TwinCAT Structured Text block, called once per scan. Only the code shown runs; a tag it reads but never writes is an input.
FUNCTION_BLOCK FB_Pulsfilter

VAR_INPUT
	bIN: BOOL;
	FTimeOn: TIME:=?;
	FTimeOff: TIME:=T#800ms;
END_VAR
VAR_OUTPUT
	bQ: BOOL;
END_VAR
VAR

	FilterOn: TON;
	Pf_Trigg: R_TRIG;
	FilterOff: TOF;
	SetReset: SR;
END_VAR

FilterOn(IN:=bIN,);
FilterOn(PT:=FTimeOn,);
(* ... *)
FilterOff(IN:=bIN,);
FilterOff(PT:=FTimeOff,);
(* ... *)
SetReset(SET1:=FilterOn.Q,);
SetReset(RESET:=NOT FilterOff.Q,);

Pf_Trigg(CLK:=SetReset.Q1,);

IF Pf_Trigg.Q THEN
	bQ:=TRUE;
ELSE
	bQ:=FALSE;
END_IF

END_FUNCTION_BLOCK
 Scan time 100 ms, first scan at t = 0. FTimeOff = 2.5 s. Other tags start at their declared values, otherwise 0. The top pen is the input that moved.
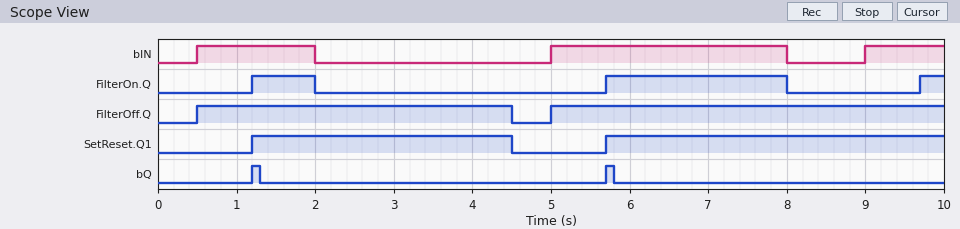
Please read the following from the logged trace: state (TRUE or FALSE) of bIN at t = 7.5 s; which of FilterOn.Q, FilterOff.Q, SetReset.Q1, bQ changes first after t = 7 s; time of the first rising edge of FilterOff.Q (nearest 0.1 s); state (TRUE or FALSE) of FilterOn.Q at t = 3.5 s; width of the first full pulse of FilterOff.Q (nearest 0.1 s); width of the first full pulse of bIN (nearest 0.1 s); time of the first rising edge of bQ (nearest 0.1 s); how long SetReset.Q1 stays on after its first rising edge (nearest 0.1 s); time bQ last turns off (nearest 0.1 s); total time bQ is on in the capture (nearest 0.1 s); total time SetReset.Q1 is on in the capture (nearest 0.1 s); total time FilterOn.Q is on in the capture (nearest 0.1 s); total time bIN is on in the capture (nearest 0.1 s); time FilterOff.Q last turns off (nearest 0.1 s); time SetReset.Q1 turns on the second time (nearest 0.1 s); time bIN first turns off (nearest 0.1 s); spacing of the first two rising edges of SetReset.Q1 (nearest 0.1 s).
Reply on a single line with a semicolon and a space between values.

TRUE; FilterOn.Q; 0.5 s; FALSE; 4.0 s; 1.5 s; 1.2 s; 3.3 s; 5.8 s; 0.2 s; 7.6 s; 3.4 s; 5.5 s; 4.5 s; 5.7 s; 2.0 s; 4.5 s
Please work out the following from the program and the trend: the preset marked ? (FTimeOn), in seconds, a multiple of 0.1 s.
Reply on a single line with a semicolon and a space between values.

0.7 s
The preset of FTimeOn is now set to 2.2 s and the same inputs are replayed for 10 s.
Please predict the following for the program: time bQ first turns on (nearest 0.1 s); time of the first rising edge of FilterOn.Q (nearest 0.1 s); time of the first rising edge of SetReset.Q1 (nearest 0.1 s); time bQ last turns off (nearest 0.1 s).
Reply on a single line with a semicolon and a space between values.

7.2 s; 7.2 s; 7.2 s; 7.3 s
